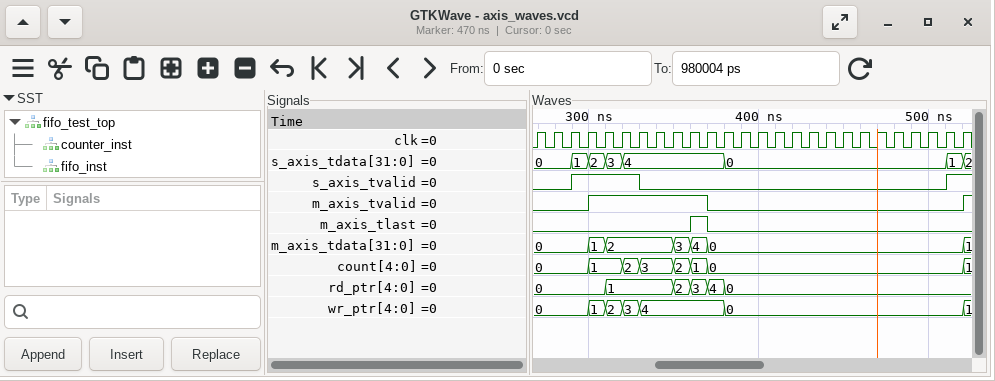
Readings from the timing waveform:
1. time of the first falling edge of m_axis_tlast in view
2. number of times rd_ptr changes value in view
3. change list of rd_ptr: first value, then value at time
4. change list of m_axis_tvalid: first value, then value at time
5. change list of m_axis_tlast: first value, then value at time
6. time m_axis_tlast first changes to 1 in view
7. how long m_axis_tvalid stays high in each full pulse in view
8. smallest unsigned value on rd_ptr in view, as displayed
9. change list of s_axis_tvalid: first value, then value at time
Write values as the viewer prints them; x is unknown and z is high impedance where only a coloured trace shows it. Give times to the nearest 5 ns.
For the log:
370 ns
5
0, 1 at 310 ns, 2 at 350 ns, 3 at 360 ns, 4 at 370 ns, 0 at 380 ns
0, 1 at 300 ns, 0 at 370 ns, 1 at 520 ns
0, 1 at 360 ns, 0 at 370 ns
360 ns
70 ns
0
0, 1 at 290 ns, 0 at 330 ns, 1 at 510 ns
